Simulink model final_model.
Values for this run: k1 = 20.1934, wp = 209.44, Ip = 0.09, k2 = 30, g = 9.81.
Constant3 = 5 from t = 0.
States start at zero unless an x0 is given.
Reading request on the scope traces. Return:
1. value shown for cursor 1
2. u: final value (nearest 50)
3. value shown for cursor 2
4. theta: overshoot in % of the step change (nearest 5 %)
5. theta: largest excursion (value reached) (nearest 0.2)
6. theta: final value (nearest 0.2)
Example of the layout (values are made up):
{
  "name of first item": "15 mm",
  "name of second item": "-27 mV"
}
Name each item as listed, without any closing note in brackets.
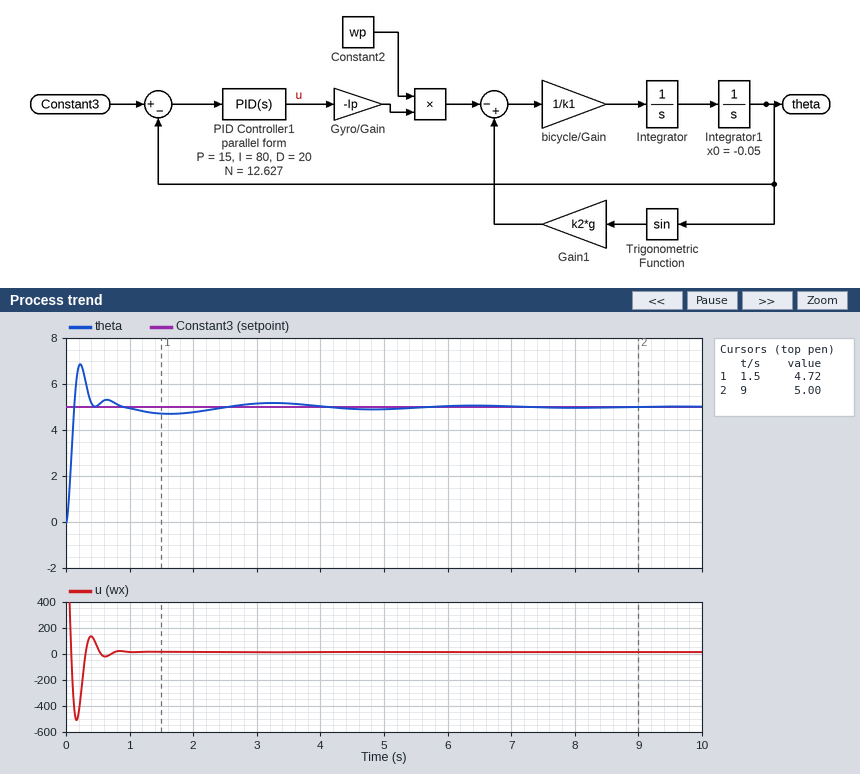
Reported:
{
  "value shown for cursor 1": "4.72",
  "u: final value": "0",
  "value shown for cursor 2": "5.00",
  "theta: overshoot in % of the step change": "35 %",
  "theta: largest excursion (value reached)": "6.8",
  "theta: final value": "5.0"
}
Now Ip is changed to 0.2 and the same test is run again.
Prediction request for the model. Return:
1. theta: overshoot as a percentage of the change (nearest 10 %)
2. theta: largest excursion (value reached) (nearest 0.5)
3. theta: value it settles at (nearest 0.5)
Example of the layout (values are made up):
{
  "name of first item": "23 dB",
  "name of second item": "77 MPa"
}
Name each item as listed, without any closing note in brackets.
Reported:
{
  "theta: overshoot as a percentage of the change": "50 %",
  "theta: largest excursion (value reached)": "7.5",
  "theta: value it settles at": "5.0"
}
